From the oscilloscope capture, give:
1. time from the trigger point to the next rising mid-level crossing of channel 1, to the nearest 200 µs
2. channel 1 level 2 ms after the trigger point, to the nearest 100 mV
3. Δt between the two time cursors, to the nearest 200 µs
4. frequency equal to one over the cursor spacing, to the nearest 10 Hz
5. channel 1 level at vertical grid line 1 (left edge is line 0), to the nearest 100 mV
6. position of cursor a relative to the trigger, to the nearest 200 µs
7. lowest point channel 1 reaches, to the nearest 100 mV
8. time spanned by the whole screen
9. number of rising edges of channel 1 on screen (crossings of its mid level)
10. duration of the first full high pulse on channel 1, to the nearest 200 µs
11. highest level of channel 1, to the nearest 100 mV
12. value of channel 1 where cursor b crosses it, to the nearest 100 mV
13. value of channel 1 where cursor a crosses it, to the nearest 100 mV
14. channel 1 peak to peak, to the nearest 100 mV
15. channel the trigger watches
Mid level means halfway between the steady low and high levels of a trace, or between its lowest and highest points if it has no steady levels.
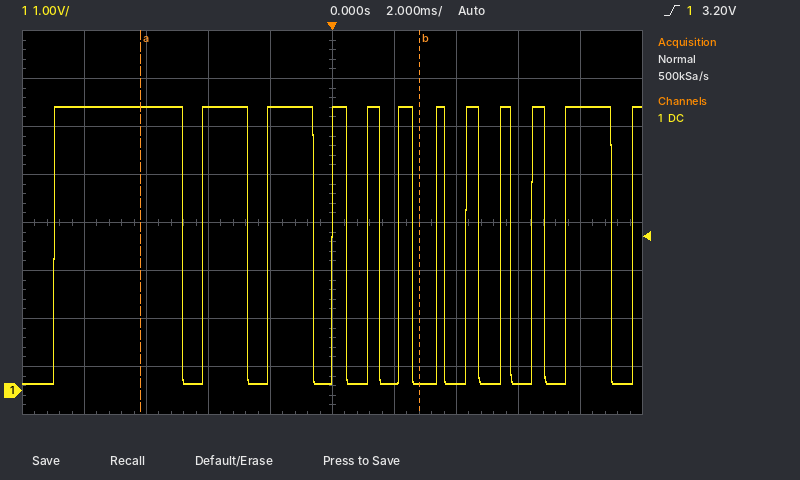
1.2 ms
100 mV
9.0 ms
110 Hz
5.9 V
-6.2 ms
100 mV
20 ms
12
4.2 ms
5.9 V
100 mV
5.9 V
5.8 V
channel 1
